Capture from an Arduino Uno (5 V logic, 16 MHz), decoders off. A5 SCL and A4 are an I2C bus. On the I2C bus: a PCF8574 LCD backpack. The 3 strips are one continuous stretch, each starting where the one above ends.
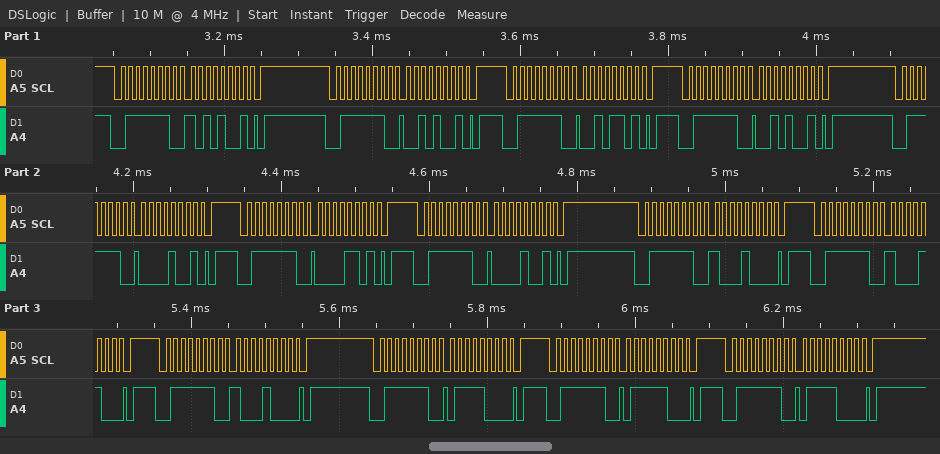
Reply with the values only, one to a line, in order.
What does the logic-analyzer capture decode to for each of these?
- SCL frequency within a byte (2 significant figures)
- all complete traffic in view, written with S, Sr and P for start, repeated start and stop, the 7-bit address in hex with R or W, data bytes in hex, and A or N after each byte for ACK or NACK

100 kHz
S 3FW A A9 A P S 3FW A 29 A P S 3FW A 2D A P S 3FW A 29 A P S 3FW A 09 A P S 3FW A 0D A P S 3FW A 09 A P S 3FW A 88 A P S 3FW A 8C A P S 3FW A 88 A P S 3FW A 78 A P S 3FW A 7C A P S 3FW A 78 A P
